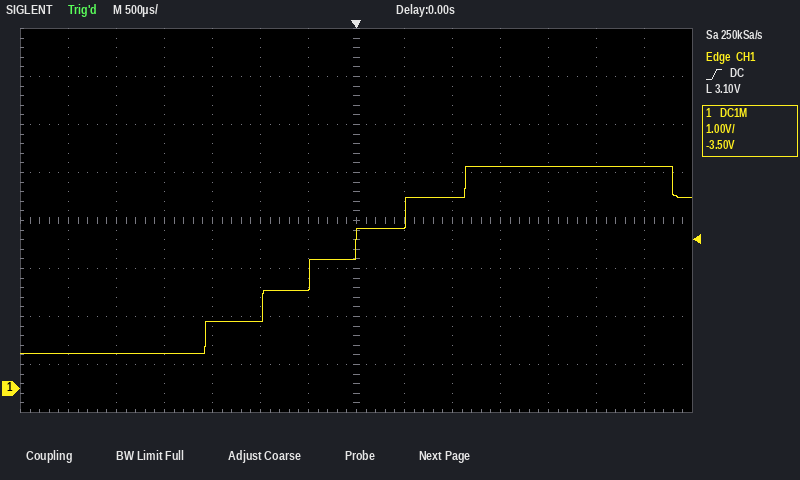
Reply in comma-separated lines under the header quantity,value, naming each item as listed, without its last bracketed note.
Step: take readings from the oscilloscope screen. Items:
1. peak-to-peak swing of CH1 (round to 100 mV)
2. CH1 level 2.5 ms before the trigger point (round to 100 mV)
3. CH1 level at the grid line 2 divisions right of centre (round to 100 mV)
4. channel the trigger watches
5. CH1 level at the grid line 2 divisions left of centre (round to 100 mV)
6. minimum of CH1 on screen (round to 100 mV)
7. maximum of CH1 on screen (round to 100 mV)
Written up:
quantity,value
peak-to-peak swing of CH1,3.9 V
CH1 level 2.5 ms before the trigger point,700 mV
CH1 level at the grid line 2 divisions right of centre,4.0 V
channel the trigger watches,CH1
CH1 level at the grid line 2 divisions left of centre,1.4 V
minimum of CH1 on screen,700 mV
maximum of CH1 on screen,4.6 V
